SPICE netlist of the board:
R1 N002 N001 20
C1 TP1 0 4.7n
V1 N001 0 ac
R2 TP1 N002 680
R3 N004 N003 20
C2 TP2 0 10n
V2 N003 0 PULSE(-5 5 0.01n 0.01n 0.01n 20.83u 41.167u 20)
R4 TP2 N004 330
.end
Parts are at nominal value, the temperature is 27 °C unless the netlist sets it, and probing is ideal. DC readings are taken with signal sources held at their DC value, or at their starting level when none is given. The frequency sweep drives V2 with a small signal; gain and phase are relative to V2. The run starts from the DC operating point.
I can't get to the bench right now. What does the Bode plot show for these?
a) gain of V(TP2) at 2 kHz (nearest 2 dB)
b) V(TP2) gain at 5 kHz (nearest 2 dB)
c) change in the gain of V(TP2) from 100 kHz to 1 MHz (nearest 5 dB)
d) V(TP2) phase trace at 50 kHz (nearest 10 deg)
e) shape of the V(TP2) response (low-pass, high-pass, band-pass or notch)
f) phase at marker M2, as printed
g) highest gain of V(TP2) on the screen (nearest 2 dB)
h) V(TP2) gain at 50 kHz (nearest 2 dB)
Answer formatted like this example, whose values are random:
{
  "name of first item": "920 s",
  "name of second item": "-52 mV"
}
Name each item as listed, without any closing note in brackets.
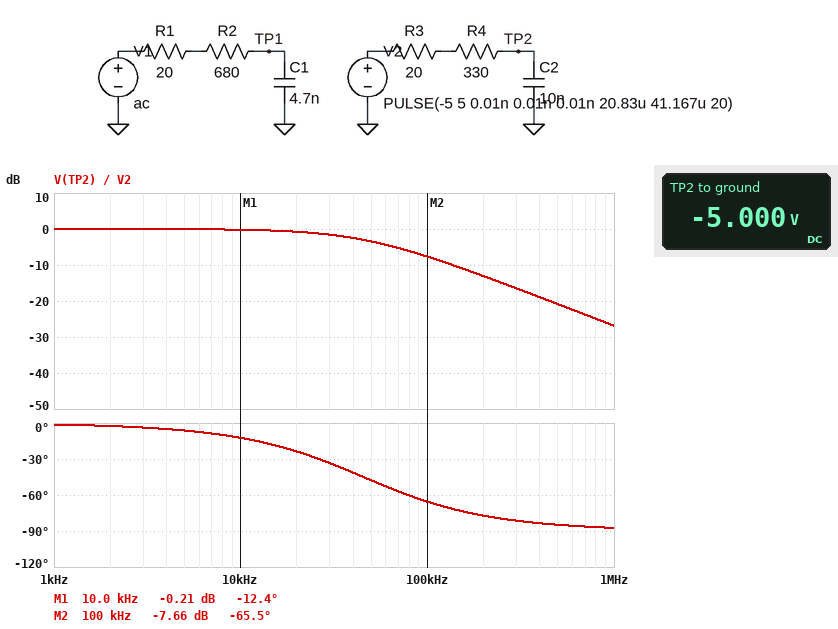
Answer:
{
  "gain of V(TP2) at 2 kHz": "0 dB",
  "V(TP2) gain at 5 kHz": "0 dB",
  "change in the gain of V(TP2) from 100 kHz to 1 MHz": "-20 dB",
  "V(TP2) phase trace at 50 kHz": "-50 deg",
  "shape of the V(TP2) response": "low-pass",
  "phase at marker M2, as printed": "-65.5 deg",
  "highest gain of V(TP2) on the screen": "0 dB",
  "V(TP2) gain at 50 kHz": "-4 dB"
}
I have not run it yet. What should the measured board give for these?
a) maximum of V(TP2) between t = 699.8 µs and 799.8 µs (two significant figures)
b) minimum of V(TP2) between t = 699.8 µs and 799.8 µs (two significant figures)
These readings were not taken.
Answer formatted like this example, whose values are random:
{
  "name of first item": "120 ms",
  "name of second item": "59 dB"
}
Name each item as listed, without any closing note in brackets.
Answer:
{
  "maximum of V(TP2) between t = 699.8 µs and 799.8 µs": "5.0 V",
  "minimum of V(TP2) between t = 699.8 µs and 799.8 µs": "-5.0 V"
}
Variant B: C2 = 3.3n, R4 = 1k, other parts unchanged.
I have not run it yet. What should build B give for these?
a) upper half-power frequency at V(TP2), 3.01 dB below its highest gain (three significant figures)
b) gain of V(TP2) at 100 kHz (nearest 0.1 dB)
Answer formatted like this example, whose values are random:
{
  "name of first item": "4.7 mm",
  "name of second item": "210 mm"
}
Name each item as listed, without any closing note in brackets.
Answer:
{
  "upper half-power frequency at V(TP2), 3.01 dB below its highest gain": "47.3 kHz",
  "gain of V(TP2) at 100 kHz": "-7.4 dB"
}
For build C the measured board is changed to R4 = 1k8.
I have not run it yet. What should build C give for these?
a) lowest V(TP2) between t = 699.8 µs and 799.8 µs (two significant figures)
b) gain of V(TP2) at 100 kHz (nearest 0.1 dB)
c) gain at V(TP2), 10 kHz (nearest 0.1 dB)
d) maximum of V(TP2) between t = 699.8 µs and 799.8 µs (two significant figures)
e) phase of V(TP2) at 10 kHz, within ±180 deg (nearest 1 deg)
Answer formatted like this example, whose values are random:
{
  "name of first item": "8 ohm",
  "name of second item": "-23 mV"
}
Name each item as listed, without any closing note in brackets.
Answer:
{
  "lowest V(TP2) between t = 699.8 µs and 799.8 µs": "-2.5 V",
  "gain of V(TP2) at 100 kHz": "-21.2 dB",
  "gain at V(TP2), 10 kHz": "-3.6 dB",
  "maximum of V(TP2) between t = 699.8 µs and 799.8 µs": "2.6 V",
  "phase of V(TP2) at 10 kHz, within ±180 deg": "-49 deg"
}
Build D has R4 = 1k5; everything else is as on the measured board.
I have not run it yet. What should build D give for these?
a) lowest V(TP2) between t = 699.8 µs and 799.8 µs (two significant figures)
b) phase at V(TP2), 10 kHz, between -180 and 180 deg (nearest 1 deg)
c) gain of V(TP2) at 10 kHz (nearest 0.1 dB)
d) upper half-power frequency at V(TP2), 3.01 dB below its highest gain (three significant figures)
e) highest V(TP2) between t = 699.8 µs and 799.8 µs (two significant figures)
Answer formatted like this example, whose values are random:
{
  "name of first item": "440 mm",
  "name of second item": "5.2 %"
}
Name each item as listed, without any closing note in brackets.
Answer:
{
  "lowest V(TP2) between t = 699.8 µs and 799.8 µs": "-2.9 V",
  "phase at V(TP2), 10 kHz, between -180 and 180 deg": "-44 deg",
  "gain of V(TP2) at 10 kHz": "-2.8 dB",
  "upper half-power frequency at V(TP2), 3.01 dB below its highest gain": "10.5 kHz",
  "highest V(TP2) between t = 699.8 µs and 799.8 µs": "3.0 V"
}
